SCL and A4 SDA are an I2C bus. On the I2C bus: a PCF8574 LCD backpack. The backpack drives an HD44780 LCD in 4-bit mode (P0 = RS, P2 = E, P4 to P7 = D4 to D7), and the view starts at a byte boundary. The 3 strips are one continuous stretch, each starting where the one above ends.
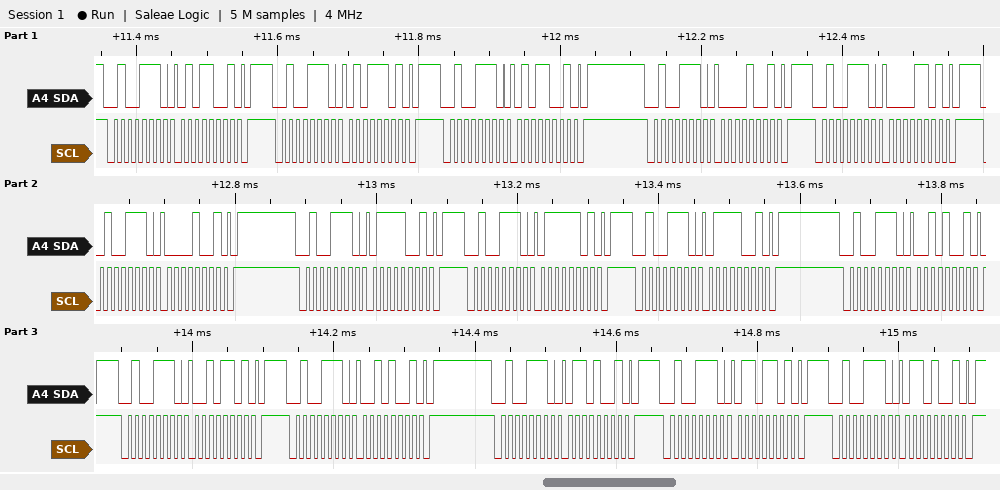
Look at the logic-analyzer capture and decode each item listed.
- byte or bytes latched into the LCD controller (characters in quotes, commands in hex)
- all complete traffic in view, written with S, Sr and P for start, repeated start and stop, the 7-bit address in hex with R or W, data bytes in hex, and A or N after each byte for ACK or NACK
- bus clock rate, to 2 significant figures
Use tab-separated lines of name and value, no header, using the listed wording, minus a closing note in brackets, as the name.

byte or bytes latched into the LCD controller	'P' 'r'
all complete traffic in view, written with S, Sr and P for start, repeated start and stop, the 7-bit address in hex with R or W, data bytes in hex, and A or N after each byte for ACK or NACK	S 27W A 59 A P S 27W A 5D A P S 27W A 59 A P S 27W A 09 A P S 27W A 0D A P S 27W A 09 A P S 27W A 79 A P S 27W A 7D A P S 27W A 79 A P S 27W A 29 A P S 27W A 2D A P S 27W A 29 A P S 27W A 69 A P S 27W A 6D A P S 27W A 69 A P
bus clock rate, to 2 significant figures	100 kHz
